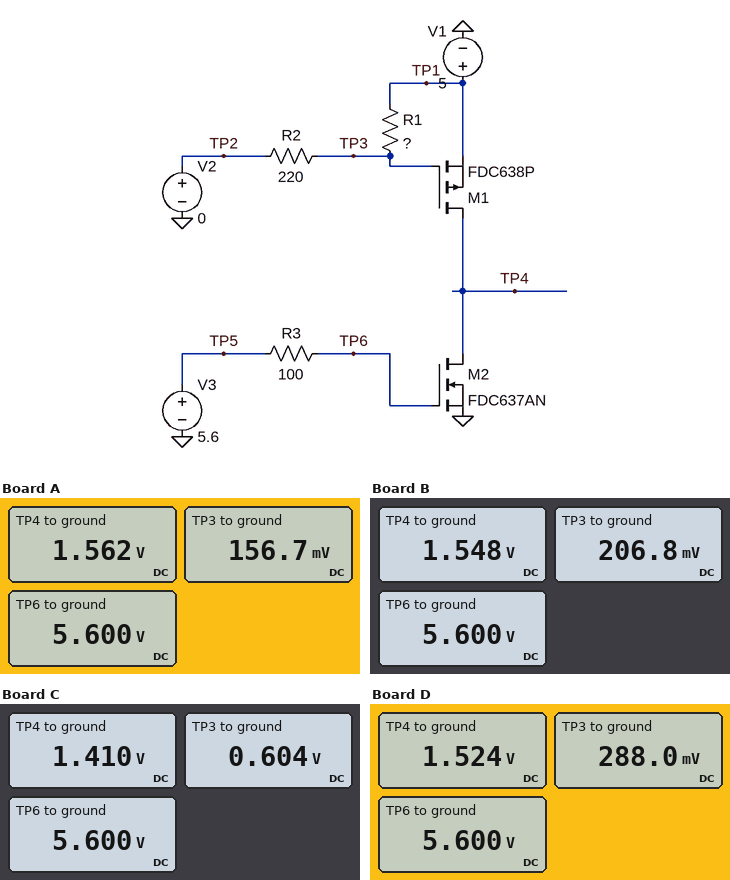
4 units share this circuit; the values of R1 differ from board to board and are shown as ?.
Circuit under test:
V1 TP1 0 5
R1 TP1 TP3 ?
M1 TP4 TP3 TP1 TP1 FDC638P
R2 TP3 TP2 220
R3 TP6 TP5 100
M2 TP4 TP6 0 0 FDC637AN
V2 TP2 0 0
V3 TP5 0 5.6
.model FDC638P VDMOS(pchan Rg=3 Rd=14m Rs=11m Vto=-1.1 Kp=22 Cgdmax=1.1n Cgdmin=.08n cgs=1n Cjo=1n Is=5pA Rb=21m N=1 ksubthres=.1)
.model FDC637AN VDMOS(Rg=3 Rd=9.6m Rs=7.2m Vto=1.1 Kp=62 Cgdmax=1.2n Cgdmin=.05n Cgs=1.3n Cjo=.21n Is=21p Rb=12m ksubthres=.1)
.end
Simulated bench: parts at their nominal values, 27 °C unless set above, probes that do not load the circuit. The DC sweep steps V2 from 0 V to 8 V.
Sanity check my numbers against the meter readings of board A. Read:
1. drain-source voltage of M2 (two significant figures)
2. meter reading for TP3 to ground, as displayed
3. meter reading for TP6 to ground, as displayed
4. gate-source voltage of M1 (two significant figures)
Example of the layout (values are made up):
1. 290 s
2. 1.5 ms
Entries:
1. 1.6 V
2. 156.7 mV
3. 5.600 V
4. -4.8 V
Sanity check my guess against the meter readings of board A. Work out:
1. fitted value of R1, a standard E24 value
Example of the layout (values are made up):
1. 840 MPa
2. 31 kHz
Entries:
1. 6.8 kΩ
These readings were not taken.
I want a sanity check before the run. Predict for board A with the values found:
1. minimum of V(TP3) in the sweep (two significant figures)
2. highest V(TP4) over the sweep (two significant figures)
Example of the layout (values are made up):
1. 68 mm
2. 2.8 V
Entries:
1. 160 mV
2. 1.6 V
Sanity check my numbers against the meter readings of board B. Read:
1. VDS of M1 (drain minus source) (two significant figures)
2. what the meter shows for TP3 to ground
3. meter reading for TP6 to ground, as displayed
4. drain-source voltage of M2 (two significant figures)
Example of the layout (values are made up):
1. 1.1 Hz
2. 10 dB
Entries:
1. -3.5 V
2. 206.8 mV
3. 5.600 V
4. 1.5 V
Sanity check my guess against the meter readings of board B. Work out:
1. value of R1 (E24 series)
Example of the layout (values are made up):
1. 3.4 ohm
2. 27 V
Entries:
1. 5.1 kΩ
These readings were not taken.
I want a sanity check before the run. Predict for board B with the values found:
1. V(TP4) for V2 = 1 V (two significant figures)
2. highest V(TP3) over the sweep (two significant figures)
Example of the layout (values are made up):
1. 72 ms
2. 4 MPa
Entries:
1. 1.1 V
2. 7.9 V
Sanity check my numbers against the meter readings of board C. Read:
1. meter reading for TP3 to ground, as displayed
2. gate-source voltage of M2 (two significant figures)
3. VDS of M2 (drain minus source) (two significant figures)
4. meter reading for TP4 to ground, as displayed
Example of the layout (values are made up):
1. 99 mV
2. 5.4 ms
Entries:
1. 0.604 V
2. 5.6 V
3. 1.4 V
4. 1.410 V
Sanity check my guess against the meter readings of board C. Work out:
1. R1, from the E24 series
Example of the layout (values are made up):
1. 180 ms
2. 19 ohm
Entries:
1. 1.6 kΩ
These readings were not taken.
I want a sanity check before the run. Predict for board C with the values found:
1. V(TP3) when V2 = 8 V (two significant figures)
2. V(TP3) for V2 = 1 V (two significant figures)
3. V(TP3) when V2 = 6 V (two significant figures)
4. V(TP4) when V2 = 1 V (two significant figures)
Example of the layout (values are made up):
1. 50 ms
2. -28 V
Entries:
1. 7.6 V
2. 1.5 V
3. 5.9 V
4. 870 mV
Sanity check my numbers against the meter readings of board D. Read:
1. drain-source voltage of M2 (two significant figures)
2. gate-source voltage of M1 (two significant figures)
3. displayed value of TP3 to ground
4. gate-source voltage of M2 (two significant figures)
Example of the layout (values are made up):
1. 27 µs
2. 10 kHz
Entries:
1. 1.5 V
2. -4.7 V
3. 288.0 mV
4. 5.6 V
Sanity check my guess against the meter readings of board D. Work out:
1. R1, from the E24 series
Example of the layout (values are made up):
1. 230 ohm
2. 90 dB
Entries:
1. 3.6 kΩ
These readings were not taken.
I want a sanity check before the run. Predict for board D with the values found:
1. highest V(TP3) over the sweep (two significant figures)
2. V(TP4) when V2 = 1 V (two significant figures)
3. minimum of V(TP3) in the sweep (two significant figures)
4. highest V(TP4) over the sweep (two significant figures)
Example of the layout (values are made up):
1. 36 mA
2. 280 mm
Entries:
1. 7.8 V
2. 1.0 V
3. 290 mV
4. 1.5 V
